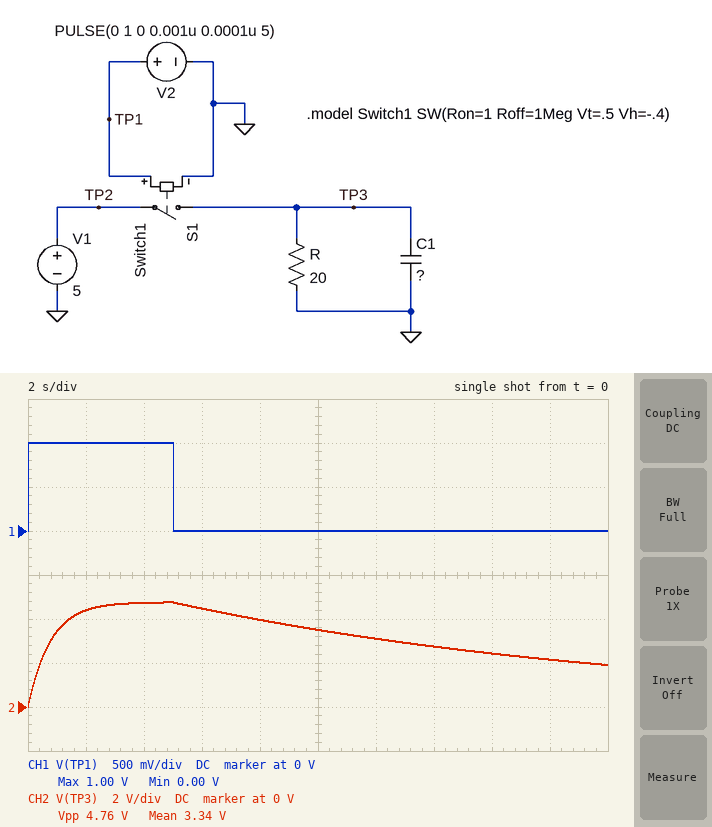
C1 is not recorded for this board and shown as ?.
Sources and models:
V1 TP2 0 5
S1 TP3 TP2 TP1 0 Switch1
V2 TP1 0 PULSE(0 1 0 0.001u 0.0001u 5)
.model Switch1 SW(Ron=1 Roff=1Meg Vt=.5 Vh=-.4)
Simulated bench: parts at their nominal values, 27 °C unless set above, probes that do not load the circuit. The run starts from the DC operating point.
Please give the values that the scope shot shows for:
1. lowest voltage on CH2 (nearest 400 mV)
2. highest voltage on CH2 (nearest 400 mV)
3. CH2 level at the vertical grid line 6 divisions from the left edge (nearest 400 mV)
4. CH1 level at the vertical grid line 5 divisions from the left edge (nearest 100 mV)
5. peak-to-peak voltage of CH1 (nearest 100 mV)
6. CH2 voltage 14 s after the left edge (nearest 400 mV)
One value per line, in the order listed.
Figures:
0 V
4.8 V
3.2 V
0 V
1.0 V
2.8 V
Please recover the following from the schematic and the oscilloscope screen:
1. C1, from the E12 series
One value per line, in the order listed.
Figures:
820 mF
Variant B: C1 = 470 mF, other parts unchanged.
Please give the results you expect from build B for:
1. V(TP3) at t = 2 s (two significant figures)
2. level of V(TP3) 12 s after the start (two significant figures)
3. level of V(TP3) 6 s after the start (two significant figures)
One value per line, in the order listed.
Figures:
4.7 V
2.3 V
4.3 V
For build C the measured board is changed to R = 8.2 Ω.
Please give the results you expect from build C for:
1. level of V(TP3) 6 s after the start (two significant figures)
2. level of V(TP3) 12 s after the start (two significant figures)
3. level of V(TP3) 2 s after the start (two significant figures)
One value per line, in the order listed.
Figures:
3.8 V
1.6 V
4.2 V
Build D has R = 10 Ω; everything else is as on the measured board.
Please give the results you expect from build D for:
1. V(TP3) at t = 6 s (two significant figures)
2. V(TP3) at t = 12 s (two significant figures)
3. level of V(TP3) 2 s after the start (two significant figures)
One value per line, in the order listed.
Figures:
4.0 V
1.9 V
4.2 V
